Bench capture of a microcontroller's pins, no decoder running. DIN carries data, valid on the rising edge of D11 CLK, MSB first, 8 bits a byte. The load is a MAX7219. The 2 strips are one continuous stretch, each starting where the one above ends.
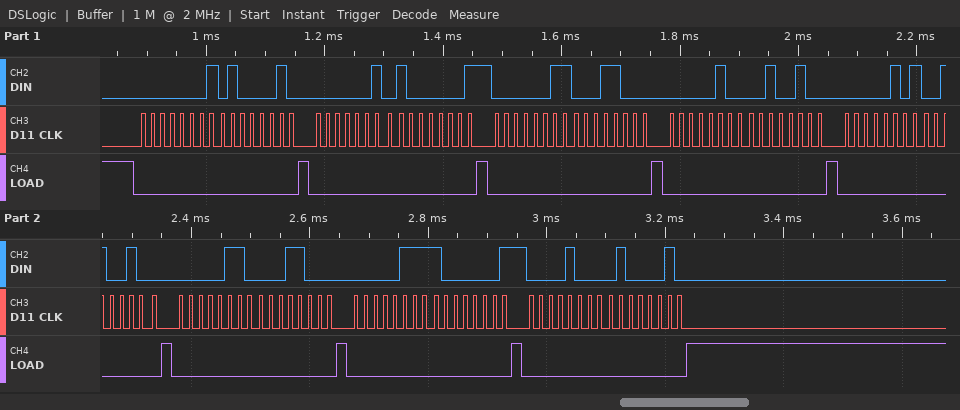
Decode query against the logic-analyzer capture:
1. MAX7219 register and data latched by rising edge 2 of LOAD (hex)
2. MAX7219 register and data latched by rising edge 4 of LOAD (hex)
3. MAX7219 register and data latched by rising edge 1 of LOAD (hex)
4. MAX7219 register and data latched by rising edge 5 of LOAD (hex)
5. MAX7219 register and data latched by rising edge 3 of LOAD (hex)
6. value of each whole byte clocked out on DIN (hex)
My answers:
register 0x2, data 0x81
register 0x4, data 0x24
register 0x1, data 0x42
register 0x5, data 0x24
register 0x3, data 0x18
01 42 02 81 03 18 04 24 05 24 06 18 07 81 08 42
